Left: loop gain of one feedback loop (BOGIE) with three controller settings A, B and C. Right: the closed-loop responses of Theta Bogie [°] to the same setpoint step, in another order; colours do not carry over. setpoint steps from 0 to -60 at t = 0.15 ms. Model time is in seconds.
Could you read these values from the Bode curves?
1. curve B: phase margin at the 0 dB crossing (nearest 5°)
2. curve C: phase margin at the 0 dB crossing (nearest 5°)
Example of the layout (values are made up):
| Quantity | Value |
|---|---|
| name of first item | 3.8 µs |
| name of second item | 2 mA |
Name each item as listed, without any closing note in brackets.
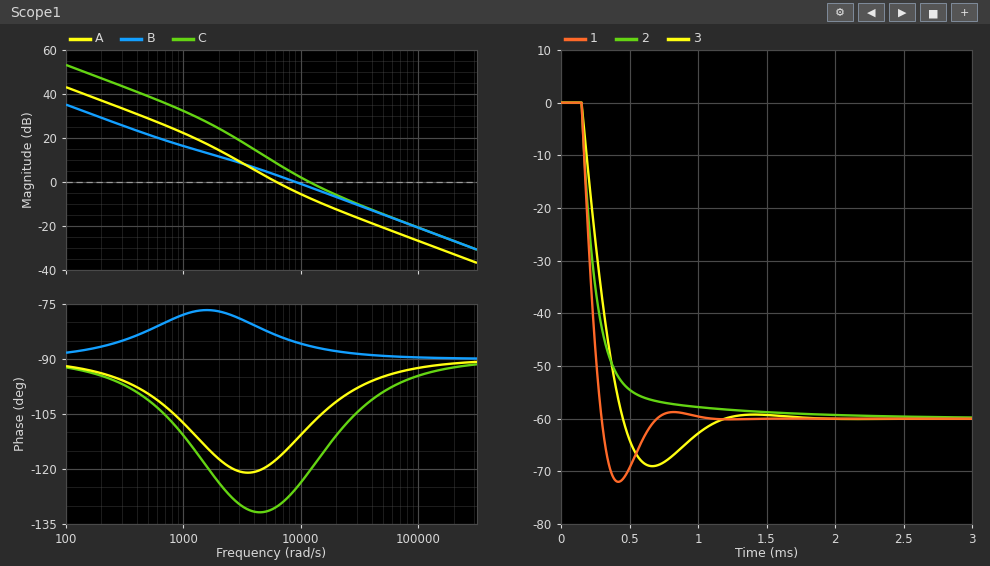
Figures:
| Quantity | Value |
|---|---|
| curve B: phase margin at the 0 dB crossing | 95° |
| curve C: phase margin at the 0 dB crossing | 60° |
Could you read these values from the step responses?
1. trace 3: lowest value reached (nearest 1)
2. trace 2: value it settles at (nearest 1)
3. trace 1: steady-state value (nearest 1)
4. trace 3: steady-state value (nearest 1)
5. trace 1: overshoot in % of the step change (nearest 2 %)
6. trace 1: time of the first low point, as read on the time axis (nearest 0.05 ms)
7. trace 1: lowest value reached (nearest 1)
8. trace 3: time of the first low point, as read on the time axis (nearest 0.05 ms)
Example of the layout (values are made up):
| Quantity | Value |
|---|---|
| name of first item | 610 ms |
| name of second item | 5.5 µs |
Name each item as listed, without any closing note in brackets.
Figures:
| Quantity | Value |
|---|---|
| trace 3: lowest value reached | -69 |
| trace 2: value it settles at | -60 |
| trace 1: steady-state value | -60 |
| trace 3: steady-state value | -60 |
| trace 1: overshoot in % of the step change | 20 % |
| trace 1: time of the first low point, as read on the time axis | 0.40 ms |
| trace 1: lowest value reached | -72 |
| trace 3: time of the first low point, as read on the time axis | 0.65 ms |
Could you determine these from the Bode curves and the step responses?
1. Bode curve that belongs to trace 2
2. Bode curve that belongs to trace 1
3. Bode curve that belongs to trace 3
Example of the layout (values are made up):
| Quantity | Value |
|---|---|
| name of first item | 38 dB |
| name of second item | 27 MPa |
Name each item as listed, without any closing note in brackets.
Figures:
| Quantity | Value |
|---|---|
| Bode curve that belongs to trace 2 | B |
| Bode curve that belongs to trace 1 | C |
| Bode curve that belongs to trace 3 | A |
